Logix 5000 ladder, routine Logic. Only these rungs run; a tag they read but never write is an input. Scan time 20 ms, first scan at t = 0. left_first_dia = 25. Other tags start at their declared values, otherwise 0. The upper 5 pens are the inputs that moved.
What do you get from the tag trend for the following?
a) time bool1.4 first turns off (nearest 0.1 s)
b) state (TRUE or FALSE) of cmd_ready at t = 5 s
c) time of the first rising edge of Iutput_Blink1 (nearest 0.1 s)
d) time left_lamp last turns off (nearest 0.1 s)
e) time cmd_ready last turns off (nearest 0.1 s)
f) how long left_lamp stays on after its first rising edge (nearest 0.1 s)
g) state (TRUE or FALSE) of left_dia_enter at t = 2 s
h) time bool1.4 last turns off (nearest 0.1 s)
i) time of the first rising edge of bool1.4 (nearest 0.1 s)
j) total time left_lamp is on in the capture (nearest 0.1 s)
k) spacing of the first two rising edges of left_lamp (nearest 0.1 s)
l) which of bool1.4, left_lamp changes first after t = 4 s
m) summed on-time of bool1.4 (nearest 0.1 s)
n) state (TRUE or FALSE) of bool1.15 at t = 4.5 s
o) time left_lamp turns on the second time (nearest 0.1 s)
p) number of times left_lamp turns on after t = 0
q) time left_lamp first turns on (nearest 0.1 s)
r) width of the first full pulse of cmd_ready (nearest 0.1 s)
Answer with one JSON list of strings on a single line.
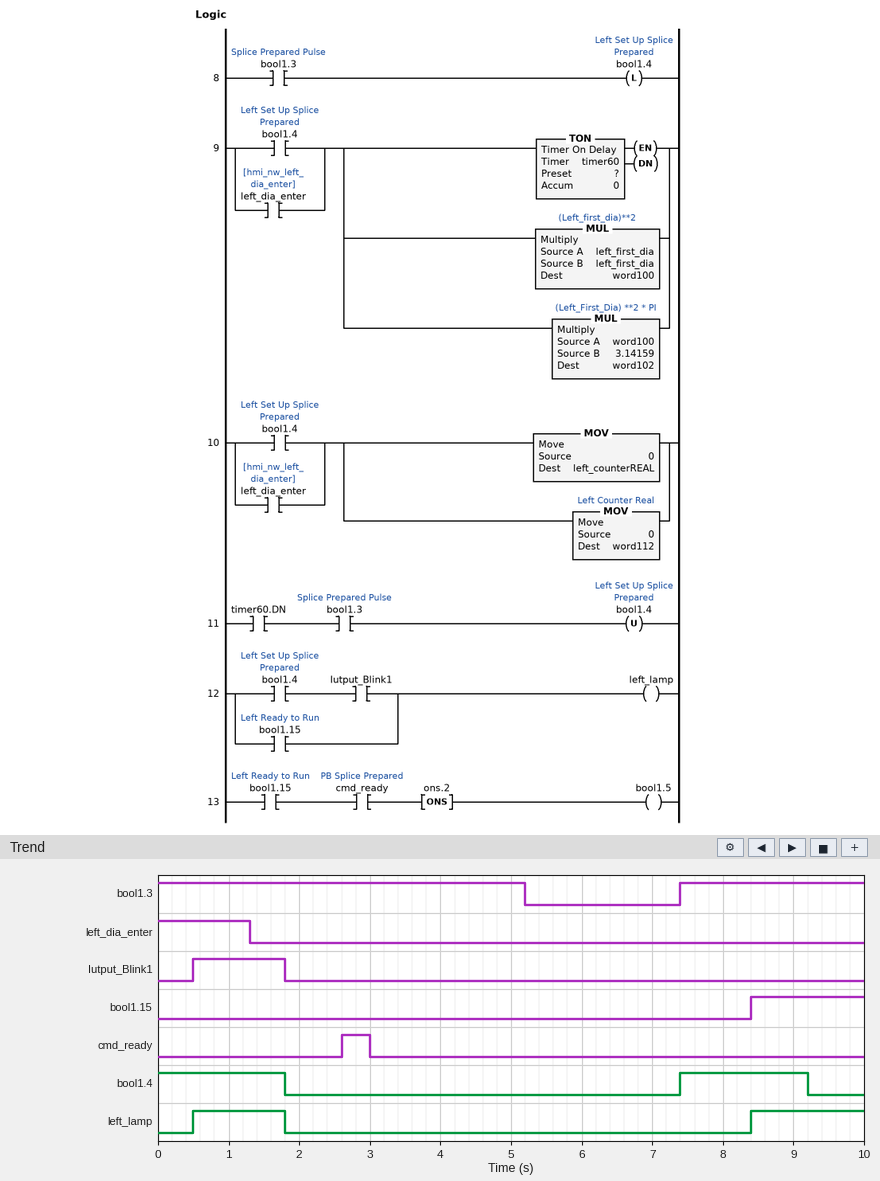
["1.8 s", "FALSE", "0.5 s", "1.8 s", "3.0 s", "1.3 s", "FALSE", "9.2 s", "7.4 s", "2.9 s", "7.9 s", "bool1.4", "3.6 s", "FALSE", "8.4 s", "2", "0.5 s", "0.4 s"]
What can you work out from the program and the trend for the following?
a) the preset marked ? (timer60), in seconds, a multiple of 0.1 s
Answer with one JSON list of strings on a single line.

["1.8 s"]
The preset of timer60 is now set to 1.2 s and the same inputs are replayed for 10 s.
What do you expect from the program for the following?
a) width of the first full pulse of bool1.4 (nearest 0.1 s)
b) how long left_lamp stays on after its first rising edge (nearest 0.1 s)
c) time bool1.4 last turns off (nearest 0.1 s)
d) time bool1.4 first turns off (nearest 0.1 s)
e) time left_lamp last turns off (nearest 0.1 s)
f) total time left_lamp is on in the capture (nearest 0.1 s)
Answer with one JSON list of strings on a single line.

["1.2 s", "0.7 s", "8.6 s", "1.2 s", "1.2 s", "2.3 s"]
